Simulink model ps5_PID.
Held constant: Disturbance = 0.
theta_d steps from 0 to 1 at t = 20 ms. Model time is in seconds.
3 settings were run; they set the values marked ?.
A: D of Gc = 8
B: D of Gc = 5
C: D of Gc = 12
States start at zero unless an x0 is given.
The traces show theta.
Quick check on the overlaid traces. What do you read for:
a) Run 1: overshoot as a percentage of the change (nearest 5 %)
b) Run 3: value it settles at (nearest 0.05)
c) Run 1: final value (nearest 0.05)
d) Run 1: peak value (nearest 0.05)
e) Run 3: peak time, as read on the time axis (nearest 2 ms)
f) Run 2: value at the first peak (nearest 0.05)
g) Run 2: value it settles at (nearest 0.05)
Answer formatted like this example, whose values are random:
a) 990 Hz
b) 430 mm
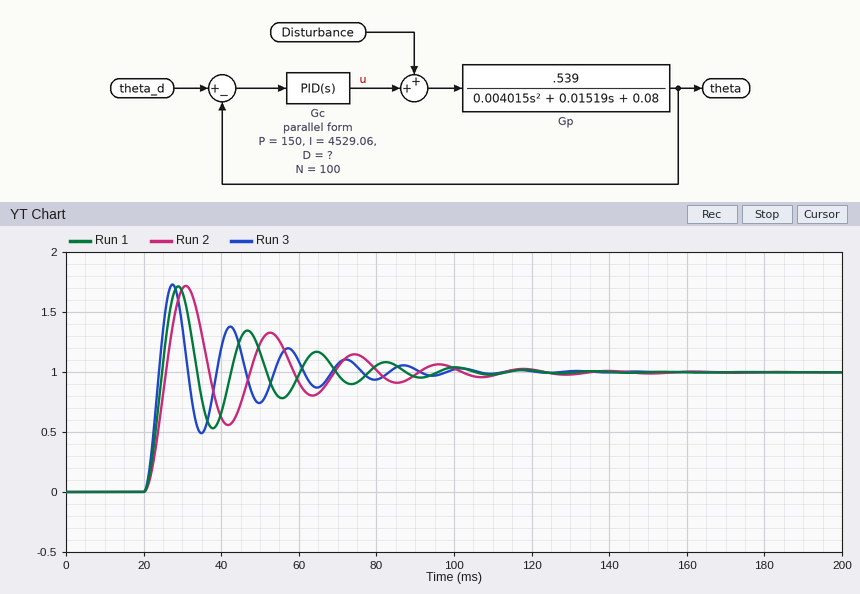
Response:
a) 70 %
b) 1.00
c) 1.00
d) 1.70
e) 28 ms
f) 1.70
g) 1.00
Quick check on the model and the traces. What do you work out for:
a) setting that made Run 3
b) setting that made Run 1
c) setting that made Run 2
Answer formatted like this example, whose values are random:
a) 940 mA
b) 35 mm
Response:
a) C
b) A
c) B
